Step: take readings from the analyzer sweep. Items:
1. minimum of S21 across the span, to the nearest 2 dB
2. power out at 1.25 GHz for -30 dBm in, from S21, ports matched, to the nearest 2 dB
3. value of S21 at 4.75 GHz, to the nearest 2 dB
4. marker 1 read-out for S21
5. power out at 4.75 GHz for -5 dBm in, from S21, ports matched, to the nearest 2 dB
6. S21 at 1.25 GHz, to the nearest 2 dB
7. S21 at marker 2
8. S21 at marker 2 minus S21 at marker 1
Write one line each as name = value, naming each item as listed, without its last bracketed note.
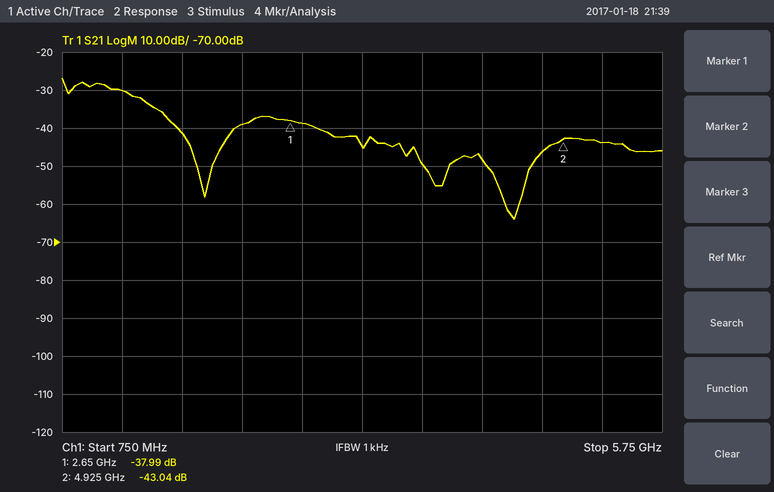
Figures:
minimum of S21 across the span, to the nearest 2 dB = -64 dB
power out at 1.25 GHz for -30 dBm in, from S21, ports matched, to the nearest 2 dB = -60 dBm
value of S21 at 4.75 GHz, to the nearest 2 dB = -46 dB
marker 1 read-out for S21 = -37.99 dB
power out at 4.75 GHz for -5 dBm in, from S21, ports matched, to the nearest 2 dB = -52 dBm
S21 at 1.25 GHz, to the nearest 2 dB = -30 dB
S21 at marker 2 = -43.04 dB
S21 at marker 2 minus S21 at marker 1 = -5.05 dB
